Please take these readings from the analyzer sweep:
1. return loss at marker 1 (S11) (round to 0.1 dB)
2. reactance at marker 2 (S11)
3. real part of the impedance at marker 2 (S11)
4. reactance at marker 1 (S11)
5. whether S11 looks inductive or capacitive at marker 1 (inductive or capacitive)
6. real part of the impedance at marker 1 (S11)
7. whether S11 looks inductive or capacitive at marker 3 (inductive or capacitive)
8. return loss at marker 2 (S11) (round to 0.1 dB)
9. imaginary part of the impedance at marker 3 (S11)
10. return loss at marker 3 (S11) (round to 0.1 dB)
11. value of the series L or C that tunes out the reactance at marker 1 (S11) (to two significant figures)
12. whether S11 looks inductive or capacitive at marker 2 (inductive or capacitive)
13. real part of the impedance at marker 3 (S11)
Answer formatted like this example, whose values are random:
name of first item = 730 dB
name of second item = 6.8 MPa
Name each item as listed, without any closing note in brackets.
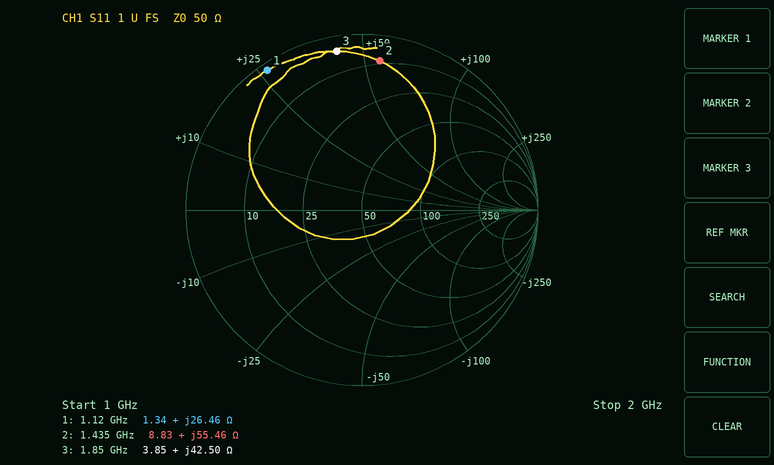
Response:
return loss at marker 1 (S11) = 0.4 dB
reactance at marker 2 = +55.46 Ω
real part of the impedance at marker 2 = 8.83 Ω
reactance at marker 1 = +26.46 Ω
whether S11 looks inductive or capacitive at marker 1 = inductive
real part of the impedance at marker 1 = 1.34 Ω
whether S11 looks inductive or capacitive at marker 3 = inductive
return loss at marker 2 (S11) = 1.4 dB
imaginary part of the impedance at marker 3 = +42.50 Ω
return loss at marker 3 (S11) = 0.8 dB
value of the series L or C that tunes out the reactance at marker 1 (S11) = 5.4 pF
whether S11 looks inductive or capacitive at marker 2 = inductive
real part of the impedance at marker 3 = 3.85 Ω
